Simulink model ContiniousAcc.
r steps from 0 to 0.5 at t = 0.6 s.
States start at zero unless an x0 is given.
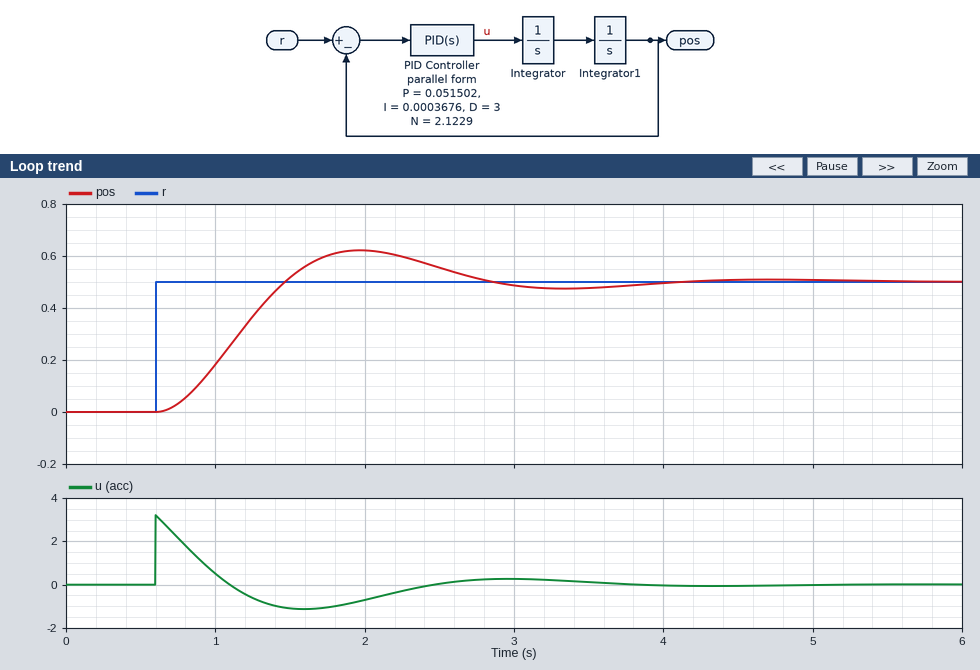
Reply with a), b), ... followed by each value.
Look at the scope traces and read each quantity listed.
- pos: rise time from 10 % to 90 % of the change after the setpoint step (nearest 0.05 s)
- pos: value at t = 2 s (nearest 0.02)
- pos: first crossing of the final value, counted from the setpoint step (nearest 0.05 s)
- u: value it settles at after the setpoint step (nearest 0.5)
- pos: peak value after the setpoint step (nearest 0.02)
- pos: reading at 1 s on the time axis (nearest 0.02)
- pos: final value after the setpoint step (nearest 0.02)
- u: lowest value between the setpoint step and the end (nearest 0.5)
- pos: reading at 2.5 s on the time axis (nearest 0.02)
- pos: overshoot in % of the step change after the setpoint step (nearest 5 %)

a) 0.60 s
b) 0.62
c) 0.85 s
d) 0.0
e) 0.62
f) 0.18
g) 0.50
h) -1.0
i) 0.56
j) 25 %
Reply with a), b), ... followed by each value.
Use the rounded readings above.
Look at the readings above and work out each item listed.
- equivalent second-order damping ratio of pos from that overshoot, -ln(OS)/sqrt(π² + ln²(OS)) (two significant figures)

a) 0.40
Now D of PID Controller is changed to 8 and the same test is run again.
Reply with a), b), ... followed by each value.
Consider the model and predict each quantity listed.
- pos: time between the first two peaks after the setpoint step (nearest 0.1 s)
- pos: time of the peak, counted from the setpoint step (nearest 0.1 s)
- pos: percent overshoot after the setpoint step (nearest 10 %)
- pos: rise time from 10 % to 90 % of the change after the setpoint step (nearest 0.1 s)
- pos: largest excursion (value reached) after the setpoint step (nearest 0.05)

a) 1.6 s
b) 0.8 s
c) 40 %
d) 0.3 s
e) 0.70
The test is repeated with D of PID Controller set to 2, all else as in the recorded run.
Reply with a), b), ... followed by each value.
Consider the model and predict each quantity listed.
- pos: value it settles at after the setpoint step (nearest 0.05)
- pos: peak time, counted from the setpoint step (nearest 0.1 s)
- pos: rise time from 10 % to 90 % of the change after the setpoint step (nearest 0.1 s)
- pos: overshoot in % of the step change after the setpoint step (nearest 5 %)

a) 0.50
b) 1.8 s
c) 0.8 s
d) 15 %
